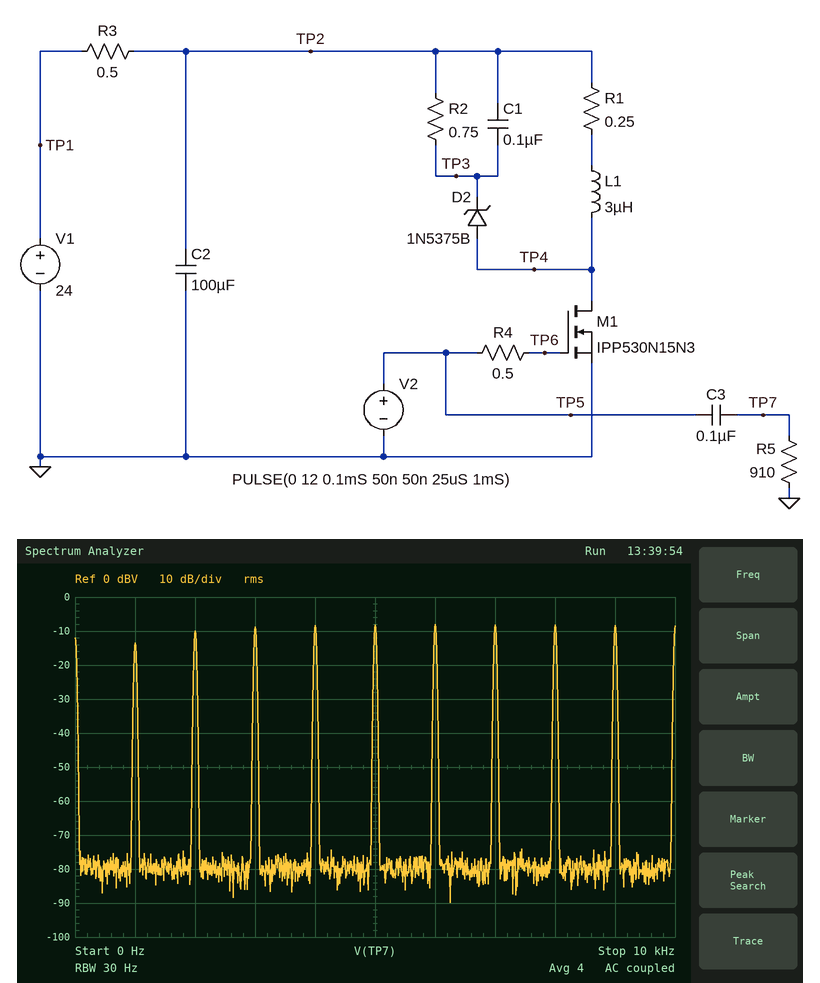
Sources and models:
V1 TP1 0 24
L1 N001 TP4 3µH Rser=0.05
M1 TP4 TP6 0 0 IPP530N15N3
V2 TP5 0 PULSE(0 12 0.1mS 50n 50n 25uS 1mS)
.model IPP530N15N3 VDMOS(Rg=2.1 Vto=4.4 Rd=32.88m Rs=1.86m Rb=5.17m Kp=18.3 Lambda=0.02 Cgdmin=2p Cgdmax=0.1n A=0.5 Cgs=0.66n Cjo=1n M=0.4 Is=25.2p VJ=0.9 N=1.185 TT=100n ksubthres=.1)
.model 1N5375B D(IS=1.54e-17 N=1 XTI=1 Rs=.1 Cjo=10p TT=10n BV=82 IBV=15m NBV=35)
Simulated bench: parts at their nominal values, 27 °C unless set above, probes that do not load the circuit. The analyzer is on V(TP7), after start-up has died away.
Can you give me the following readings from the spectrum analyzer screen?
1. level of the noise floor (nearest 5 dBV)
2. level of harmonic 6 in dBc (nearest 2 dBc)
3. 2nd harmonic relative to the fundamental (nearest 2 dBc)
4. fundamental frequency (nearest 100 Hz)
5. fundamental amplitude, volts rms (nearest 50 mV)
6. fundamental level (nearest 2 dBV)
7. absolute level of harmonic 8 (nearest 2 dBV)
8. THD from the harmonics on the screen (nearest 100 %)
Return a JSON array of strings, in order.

["-80 dBV", "6 dBc", "4 dBc", "1.0 kHz", "200 mV", "-14 dBV", "-8 dBV", "500 %"]
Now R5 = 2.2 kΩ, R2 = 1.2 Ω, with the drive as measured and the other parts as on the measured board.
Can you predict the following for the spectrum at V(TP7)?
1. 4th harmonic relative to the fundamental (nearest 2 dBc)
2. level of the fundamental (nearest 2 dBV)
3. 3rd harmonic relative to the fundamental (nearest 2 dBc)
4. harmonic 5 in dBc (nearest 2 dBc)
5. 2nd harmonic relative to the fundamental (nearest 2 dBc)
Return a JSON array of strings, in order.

["2 dBc", "-10 dBV", "2 dBc", "2 dBc", "2 dBc"]
